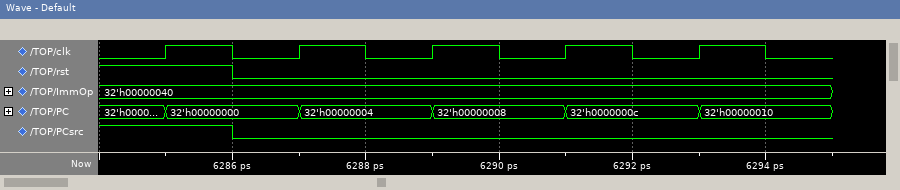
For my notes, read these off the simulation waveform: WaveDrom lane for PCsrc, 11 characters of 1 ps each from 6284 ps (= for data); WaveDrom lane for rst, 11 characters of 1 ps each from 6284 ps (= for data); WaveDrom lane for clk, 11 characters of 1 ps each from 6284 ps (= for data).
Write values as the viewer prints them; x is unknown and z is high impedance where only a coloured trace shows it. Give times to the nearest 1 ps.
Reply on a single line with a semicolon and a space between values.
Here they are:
{name: 'PCsrc', wave: '1.0........'}; {name: 'rst', wave: '1.0........'}; {name: 'clk', wave: '01010101010'}
